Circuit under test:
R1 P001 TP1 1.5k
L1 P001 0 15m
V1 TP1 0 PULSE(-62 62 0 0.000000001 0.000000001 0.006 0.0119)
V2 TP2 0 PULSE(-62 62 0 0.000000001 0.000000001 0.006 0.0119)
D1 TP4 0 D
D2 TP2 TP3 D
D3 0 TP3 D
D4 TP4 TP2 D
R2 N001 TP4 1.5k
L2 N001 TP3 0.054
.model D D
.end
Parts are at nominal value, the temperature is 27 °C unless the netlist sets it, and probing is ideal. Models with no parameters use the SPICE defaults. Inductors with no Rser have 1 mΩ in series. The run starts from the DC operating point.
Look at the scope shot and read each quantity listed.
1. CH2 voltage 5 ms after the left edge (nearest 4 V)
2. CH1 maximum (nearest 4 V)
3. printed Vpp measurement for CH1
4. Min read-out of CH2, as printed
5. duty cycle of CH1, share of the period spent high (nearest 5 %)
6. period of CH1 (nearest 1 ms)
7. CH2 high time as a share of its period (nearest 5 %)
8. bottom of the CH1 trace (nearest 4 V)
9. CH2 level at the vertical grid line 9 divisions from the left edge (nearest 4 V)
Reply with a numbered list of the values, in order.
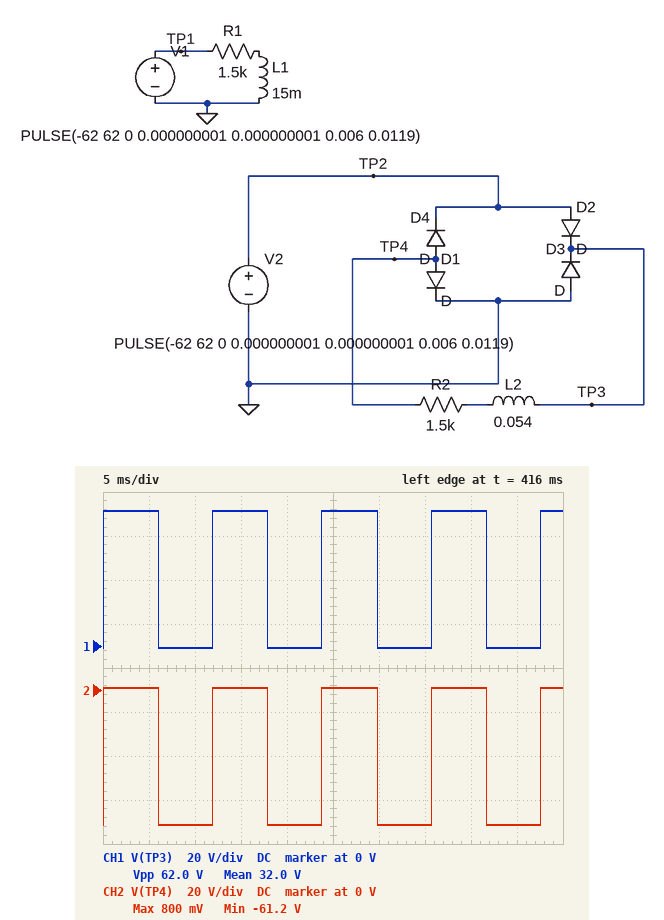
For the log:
1. 0 V
2. 60 V
3. 62.0 V
4. -61.2 V
5. 50 %
6. 12 ms
7. 50 %
8. 0 V
9. -60 V
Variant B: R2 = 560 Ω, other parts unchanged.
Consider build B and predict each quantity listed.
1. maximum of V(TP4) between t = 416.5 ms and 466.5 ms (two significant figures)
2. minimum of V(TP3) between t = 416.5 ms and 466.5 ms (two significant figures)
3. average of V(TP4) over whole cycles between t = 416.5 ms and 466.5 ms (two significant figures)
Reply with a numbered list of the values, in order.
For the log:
1. 780 mV
2. -780 mV
3. -30 V
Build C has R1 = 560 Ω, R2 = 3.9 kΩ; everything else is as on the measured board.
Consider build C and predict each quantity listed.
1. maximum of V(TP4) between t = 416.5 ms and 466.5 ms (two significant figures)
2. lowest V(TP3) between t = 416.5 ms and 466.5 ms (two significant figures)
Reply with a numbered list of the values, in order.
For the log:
1. 730 mV
2. -730 mV
